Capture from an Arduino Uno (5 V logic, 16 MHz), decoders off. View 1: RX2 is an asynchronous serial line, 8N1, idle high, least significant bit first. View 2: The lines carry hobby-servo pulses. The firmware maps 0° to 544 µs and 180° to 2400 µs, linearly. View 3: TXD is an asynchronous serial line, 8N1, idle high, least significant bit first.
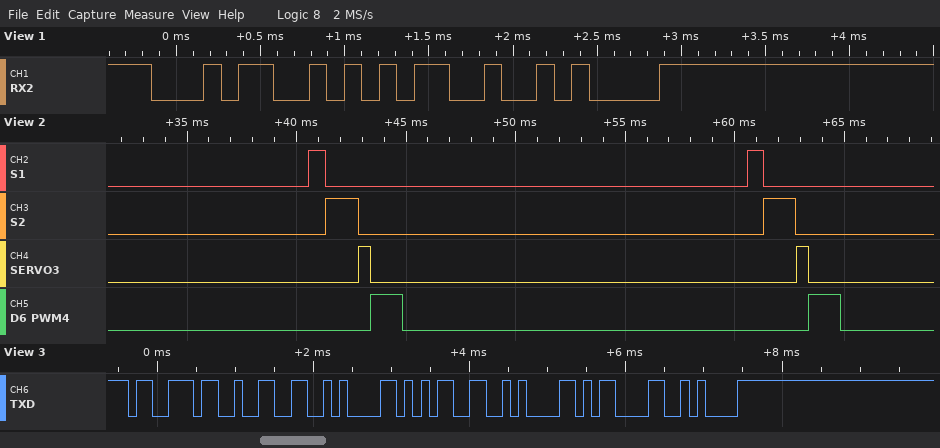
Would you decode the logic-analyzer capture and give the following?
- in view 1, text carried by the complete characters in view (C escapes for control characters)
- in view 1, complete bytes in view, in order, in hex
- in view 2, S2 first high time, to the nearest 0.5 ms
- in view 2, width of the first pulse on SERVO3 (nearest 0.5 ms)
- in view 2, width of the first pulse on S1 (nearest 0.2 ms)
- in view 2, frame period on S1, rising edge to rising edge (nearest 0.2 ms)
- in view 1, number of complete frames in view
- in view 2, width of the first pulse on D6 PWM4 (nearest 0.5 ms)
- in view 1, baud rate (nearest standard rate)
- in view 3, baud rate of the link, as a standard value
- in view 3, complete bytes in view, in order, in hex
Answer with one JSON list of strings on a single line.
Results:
["\"45\\n\"", "0x34 0x35 0x0A", "1.5 ms", "0.5 ms", "0.8 ms", "20.0 ms", "3", "1.5 ms", "9600 baud", "9600 baud", "0x73 0x32 0x0A 0x35 0x0A 0x0D 0x0A"]
